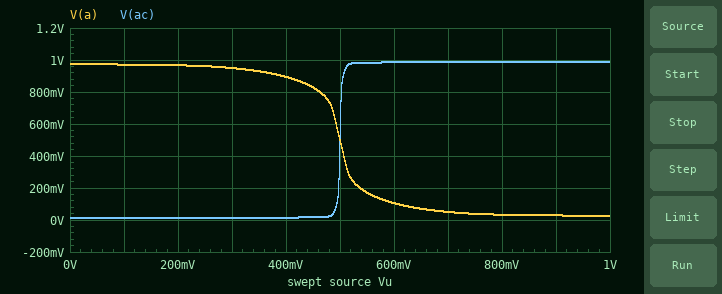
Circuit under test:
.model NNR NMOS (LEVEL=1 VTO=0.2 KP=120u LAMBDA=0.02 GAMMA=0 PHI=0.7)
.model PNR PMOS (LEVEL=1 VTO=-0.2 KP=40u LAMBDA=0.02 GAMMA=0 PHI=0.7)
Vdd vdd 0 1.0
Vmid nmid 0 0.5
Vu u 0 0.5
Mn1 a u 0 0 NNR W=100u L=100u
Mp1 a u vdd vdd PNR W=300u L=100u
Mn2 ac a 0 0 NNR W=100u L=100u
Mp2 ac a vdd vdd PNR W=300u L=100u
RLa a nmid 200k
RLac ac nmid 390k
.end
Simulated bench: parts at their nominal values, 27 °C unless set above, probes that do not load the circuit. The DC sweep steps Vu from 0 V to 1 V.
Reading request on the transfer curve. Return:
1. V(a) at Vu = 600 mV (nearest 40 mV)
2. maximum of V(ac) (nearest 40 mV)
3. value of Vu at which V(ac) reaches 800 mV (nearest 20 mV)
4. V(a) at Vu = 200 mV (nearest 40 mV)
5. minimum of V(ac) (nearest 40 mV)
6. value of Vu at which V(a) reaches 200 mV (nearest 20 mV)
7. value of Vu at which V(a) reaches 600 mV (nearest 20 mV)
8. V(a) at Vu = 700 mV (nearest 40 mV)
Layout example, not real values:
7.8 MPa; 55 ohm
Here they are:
120 mV; 1.00 V; 500 mV; 960 mV; 0 V; 540 mV; 500 mV; 40 mV
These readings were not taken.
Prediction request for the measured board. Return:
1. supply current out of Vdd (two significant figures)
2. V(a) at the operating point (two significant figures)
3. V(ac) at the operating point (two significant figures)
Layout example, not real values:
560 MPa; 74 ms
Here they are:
11 µA; 500 mV; 500 mV
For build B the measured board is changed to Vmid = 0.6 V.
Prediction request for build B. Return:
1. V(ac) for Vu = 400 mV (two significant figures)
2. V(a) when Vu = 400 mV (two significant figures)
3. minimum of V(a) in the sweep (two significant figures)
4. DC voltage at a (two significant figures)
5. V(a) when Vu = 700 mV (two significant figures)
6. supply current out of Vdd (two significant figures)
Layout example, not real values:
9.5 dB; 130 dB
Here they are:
18 mV; 910 mV; 30 mV; 600 mV; 59 mV; 8.0 µA
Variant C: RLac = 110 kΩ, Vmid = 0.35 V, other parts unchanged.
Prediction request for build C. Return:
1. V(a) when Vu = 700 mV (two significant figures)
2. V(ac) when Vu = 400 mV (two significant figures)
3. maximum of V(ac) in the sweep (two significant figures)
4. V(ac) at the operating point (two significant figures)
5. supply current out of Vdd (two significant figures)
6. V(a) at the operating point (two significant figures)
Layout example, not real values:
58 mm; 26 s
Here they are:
38 mV; 36 mV; 940 mV; 860 mV; 12 µA; 360 mV
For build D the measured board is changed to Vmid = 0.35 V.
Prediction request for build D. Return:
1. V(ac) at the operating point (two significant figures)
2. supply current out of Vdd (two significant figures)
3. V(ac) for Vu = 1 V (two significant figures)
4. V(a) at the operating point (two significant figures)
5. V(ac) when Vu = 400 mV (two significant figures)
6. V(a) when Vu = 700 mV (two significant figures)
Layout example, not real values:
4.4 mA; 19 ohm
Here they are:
940 mV; 8.5 µA; 980 mV; 360 mV; 11 mV; 38 mV
